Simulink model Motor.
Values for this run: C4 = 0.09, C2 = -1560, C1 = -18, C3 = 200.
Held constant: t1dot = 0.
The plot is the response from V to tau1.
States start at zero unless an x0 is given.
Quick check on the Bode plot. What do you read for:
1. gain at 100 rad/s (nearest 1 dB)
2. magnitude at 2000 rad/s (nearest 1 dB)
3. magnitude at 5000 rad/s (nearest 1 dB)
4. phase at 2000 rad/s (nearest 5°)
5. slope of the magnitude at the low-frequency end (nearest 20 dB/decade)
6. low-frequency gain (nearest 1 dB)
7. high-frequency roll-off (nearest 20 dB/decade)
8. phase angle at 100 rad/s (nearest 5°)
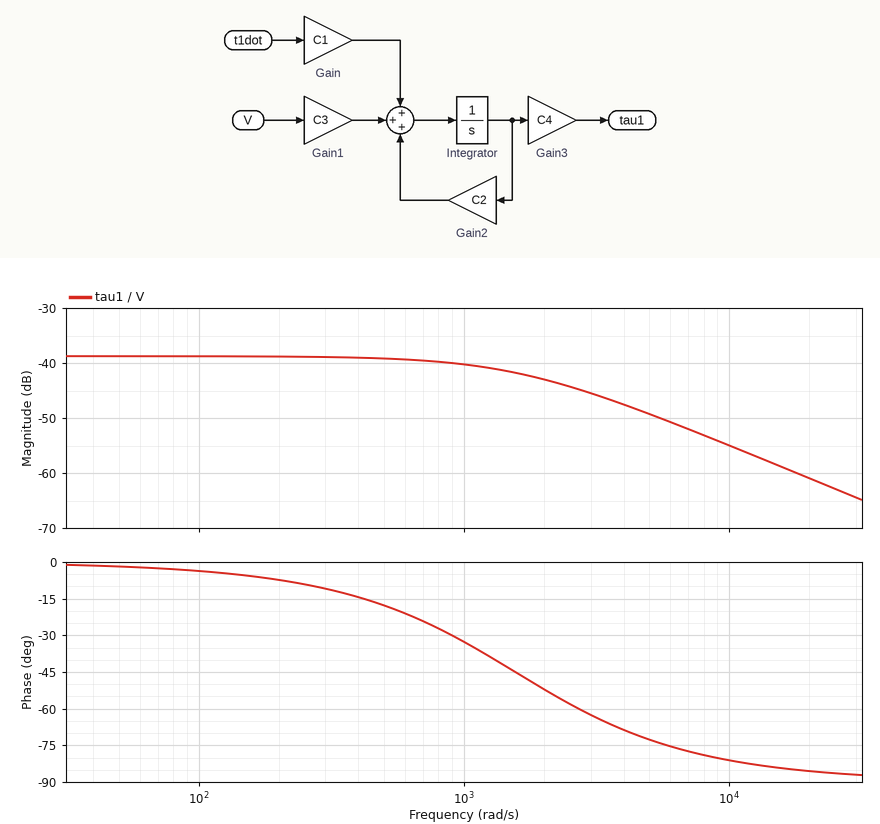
-39 dB
-43 dB
-49 dB
-50°
0 dB/decade
-39 dB
-20 dB/decade
-5°
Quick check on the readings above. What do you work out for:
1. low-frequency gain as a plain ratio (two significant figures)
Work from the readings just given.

0.011
